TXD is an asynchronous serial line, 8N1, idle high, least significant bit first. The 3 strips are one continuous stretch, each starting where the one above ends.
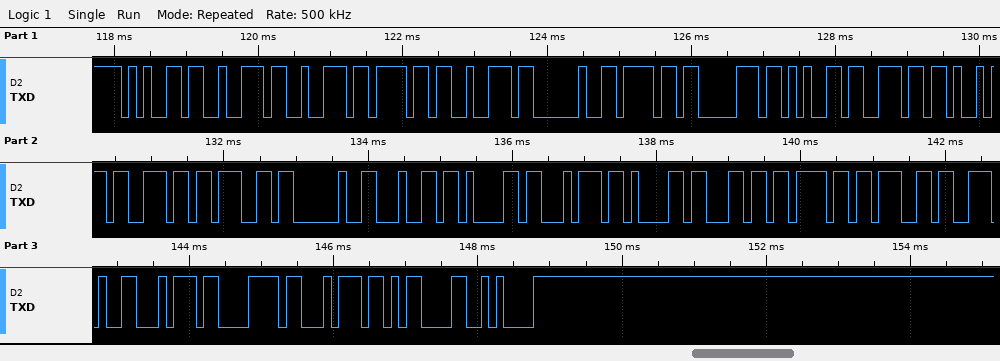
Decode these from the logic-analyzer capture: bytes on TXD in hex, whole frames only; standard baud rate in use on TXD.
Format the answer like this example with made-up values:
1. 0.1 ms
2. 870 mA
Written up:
1. 65 72 72 6F 72 20 6F 70 65 6E 69 6E 67 20 64 61 74 61 6C 6F 67 2E 74 78 74 0D 0A
2. 9600 baud
